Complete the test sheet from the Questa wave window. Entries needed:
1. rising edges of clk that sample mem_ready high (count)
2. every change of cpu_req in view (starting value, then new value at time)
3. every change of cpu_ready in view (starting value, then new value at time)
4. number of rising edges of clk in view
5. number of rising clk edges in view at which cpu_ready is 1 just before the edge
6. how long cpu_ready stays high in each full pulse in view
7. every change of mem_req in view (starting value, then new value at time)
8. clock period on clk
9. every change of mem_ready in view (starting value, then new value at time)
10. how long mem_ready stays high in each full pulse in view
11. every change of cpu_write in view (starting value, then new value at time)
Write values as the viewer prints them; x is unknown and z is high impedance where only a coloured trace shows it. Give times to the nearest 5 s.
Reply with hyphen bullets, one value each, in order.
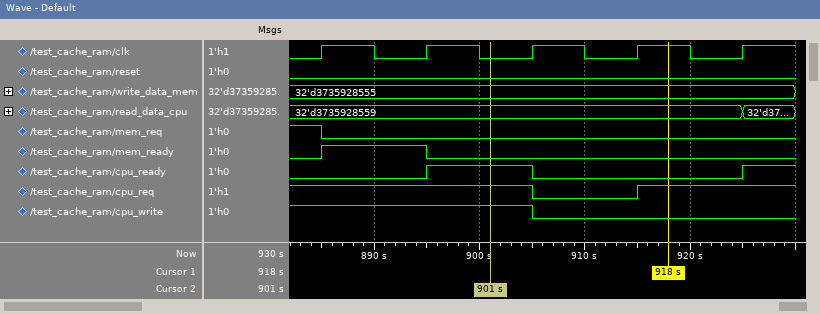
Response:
- 1
- 1, 0 at 905 s, 1 at 915 s
- 0, 1 at 895 s, 0 at 905 s, 1 at 925 s
- 5
- 1
- 10 s
- 1, 0 at 885 s
- 10 s
- 0, 1 at 885 s, 0 at 895 s
- 10 s
- 1, 0 at 905 s
